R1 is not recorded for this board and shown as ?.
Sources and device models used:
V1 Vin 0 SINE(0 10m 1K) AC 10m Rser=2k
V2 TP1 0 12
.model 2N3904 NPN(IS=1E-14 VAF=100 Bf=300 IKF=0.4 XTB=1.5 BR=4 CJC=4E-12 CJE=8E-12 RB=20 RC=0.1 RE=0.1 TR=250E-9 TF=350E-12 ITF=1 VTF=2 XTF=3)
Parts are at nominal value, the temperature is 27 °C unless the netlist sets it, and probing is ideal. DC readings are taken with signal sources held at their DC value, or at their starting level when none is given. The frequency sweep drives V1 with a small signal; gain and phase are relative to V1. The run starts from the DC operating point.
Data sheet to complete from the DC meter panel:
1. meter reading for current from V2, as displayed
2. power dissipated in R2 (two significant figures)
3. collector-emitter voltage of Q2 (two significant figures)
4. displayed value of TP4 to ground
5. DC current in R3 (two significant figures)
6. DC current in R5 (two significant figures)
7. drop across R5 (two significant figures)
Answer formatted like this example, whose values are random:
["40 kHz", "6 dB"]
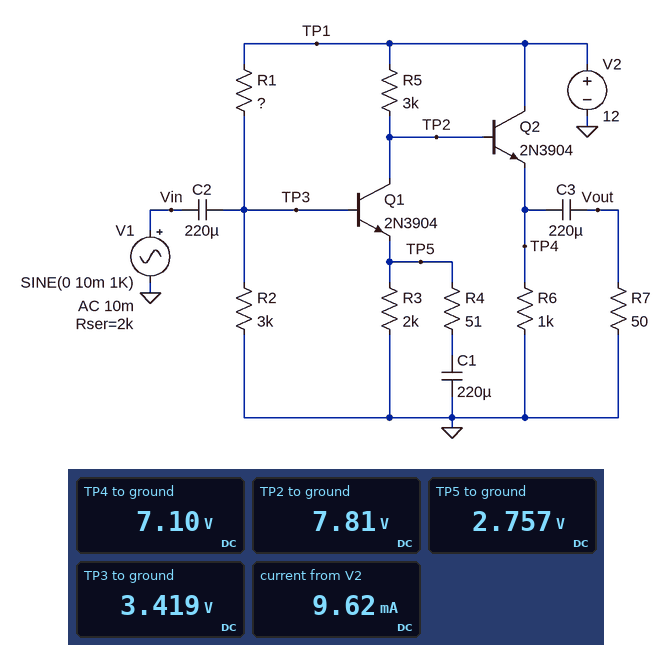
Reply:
["9.62 mA", "3.9 mW", "4.9 V", "7.10 V", "1.4 mA", "1.4 mA", "4.2 V"]
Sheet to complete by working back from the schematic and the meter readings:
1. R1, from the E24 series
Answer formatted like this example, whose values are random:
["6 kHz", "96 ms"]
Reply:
["7.5 kΩ"]
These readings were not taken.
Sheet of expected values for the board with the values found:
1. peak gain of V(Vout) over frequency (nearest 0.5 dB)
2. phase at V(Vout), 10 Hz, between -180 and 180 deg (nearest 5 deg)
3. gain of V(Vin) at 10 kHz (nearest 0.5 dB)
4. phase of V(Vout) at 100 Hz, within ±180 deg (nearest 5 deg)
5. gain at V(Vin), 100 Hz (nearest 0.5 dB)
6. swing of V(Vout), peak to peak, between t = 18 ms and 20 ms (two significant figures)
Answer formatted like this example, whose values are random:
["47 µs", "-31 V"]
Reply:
["24.5 dB", "-90 deg", "-6.0 dB", "-170 deg", "-6.0 dB", "330 mV"]
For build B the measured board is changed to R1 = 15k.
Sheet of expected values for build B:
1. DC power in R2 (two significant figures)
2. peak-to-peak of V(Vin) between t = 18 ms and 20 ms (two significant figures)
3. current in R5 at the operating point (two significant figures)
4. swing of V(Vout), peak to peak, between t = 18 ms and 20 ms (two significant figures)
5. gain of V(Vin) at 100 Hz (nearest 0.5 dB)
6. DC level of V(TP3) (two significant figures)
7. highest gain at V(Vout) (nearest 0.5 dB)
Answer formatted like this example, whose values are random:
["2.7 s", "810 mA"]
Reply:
["1.3 mW", "11 mV", "700 µA", "280 mV", "-5.5 dB", "2.0 V", "23.0 dB"]
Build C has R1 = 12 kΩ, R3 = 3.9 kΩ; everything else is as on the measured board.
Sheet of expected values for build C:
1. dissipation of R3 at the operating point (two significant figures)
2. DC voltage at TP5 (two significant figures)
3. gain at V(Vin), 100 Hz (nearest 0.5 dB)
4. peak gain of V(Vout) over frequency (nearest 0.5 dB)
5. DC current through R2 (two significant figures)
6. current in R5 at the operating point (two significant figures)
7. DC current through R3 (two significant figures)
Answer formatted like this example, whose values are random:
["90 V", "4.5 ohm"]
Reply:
["800 µW", "1.8 V", "-5.5 dB", "21.0 dB", "800 µA", "480 µA", "450 µA"]
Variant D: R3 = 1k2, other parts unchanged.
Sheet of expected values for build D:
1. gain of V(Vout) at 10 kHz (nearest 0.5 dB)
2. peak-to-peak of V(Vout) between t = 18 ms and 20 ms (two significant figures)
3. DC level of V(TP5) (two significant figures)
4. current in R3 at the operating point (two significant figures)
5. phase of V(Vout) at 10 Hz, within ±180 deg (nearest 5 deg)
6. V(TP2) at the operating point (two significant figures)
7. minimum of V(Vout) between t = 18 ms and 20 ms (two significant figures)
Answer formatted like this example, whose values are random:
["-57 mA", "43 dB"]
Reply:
["25.0 dB", "350 mV", "2.7 V", "2.3 mA", "-85 deg", "5.1 V", "-170 mV"]
